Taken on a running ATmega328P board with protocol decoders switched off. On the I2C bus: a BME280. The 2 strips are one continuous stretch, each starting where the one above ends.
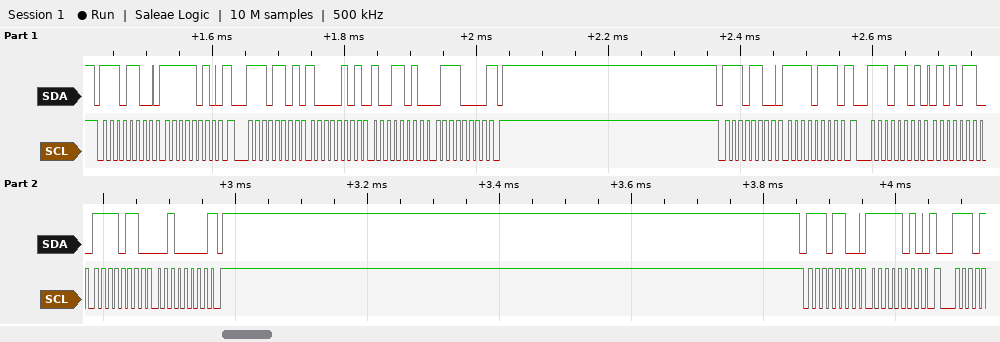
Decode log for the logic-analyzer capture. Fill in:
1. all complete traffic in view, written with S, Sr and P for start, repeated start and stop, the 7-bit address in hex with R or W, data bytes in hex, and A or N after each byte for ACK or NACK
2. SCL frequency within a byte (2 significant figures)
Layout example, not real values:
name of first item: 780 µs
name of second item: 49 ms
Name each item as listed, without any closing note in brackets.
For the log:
all complete traffic in view, written with S, Sr and P for start, repeated start and stop, the 7-bit address in hex with R or W, data bytes in hex, and A or N after each byte for ACK or NACK: S 76W A FA A Sr 76R A 85 A 9A A 70 N P S 76W A F7 A Sr 76R A 56 A F6 A 20 N P S 76W A FA A
SCL frequency within a byte: 100 kHz
